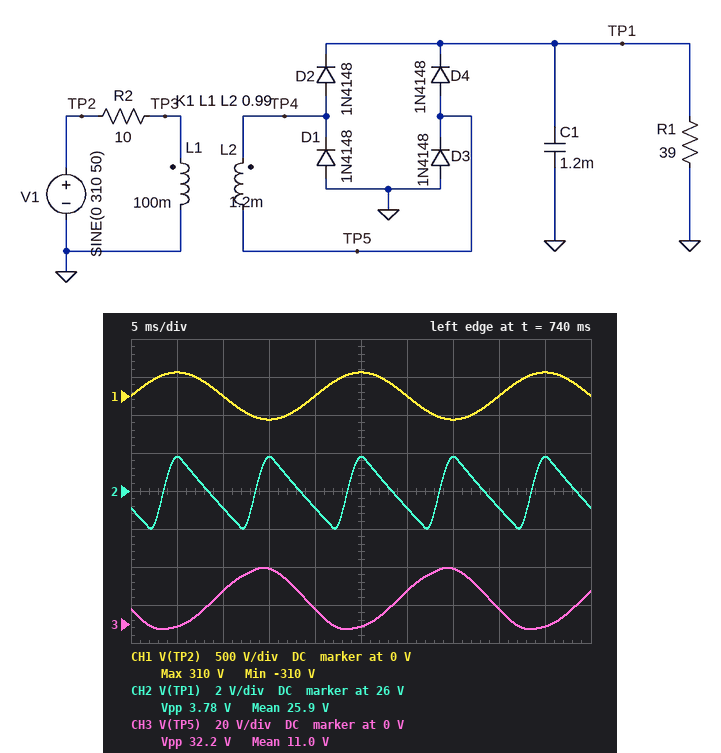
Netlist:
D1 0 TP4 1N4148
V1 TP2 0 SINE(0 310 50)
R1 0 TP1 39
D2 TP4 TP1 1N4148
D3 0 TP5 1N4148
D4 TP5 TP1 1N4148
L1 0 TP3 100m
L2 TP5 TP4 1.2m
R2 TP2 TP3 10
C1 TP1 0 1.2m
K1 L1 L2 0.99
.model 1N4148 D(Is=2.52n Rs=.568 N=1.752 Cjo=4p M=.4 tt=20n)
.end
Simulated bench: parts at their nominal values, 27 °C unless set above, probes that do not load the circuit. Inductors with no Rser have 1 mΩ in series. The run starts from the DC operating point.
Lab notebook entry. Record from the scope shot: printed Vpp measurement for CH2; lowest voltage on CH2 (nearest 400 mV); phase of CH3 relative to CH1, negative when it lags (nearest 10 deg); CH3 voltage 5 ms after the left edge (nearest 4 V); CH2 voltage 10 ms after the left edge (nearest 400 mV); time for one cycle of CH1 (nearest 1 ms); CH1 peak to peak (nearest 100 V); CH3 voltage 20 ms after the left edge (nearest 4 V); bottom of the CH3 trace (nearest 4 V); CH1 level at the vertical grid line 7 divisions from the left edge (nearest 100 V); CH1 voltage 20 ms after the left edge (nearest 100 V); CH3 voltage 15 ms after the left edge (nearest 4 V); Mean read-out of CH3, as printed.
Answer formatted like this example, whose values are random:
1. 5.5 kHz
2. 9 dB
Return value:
1. 3.78 V
2. 24.0 V
3. -160 deg
4. 0 V
5. 25.2 V
6. 20 ms
7. 600 V
8. 8 V
9. -4 V
10. -300 V
11. 0 V
12. 28 V
13. 11.0 V
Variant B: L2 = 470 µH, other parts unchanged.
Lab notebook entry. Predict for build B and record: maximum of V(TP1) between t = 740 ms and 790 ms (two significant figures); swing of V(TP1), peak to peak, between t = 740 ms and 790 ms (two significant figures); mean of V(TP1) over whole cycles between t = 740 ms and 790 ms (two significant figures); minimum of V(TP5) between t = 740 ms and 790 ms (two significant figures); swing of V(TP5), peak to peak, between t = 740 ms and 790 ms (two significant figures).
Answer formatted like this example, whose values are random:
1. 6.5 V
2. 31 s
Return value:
1. 17 V
2. 2.3 V
3. 16 V
4. -2.0 V
5. 20 V
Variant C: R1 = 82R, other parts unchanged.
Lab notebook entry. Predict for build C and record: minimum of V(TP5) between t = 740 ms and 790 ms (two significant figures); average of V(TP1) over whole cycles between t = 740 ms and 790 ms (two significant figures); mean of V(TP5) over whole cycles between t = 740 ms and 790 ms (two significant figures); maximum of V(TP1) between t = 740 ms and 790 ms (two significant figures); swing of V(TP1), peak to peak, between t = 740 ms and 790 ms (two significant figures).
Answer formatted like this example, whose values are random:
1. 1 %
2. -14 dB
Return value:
1. -2.0 V
2. 28 V
3. 14 V
4. 29 V
5. 2.1 V
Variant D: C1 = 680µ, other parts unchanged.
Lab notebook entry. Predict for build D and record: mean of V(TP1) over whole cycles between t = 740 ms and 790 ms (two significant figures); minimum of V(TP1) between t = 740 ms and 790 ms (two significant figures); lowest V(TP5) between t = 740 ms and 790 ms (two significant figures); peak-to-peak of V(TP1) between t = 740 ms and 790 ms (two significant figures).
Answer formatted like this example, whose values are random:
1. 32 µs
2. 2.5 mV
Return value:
1. 25 V
2. 22 V
3. -2.6 V
4. 6.4 V
